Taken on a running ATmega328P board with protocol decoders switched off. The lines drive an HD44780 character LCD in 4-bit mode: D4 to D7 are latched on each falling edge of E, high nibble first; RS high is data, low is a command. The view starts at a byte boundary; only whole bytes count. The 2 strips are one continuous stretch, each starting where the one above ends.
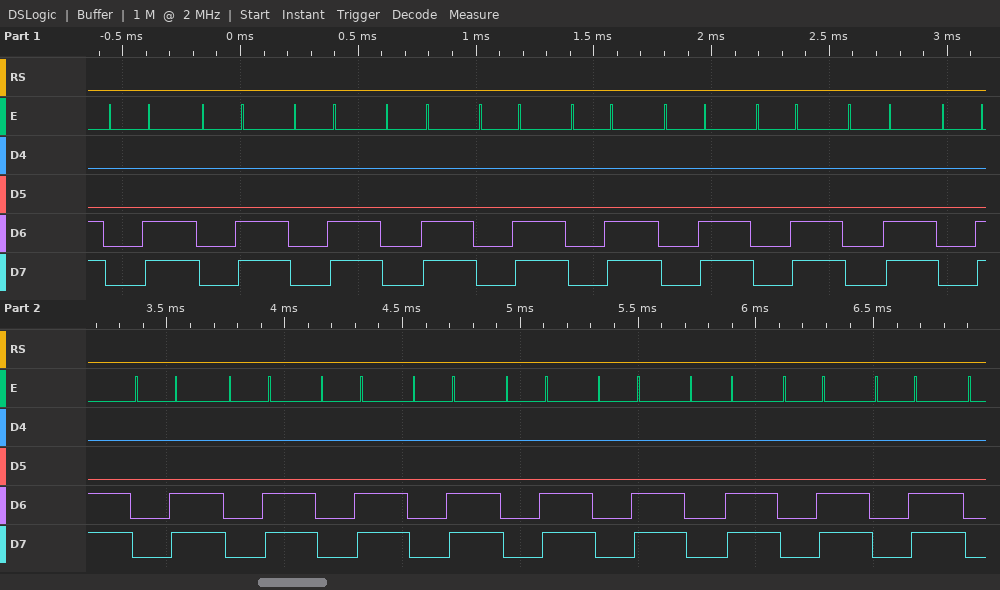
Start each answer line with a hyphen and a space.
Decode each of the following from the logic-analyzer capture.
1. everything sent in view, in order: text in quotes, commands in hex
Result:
- 0x0C 0x0C 0x0C 0x0C 0x0C 0x0C 0x0C 0x0C 0x0C 0x0C 0x0C 0x0C 0x0C 0x0C 0x0C 0x0C 0x0C 0x0C 0x0C
